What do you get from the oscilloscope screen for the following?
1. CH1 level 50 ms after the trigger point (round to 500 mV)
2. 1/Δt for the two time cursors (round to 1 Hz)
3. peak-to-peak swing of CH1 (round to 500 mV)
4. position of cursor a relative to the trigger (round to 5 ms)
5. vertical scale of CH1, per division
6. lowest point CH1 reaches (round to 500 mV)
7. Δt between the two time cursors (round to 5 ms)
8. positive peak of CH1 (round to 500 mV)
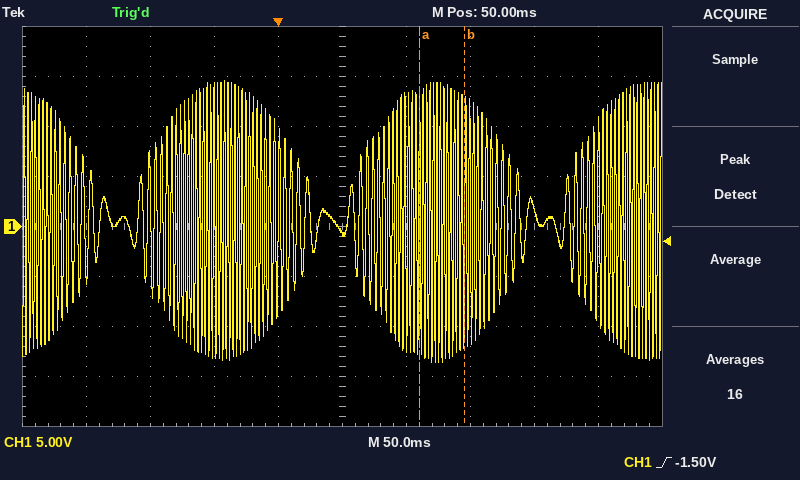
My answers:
-500 mV
29 Hz
28.0 V
+110 ms
5 V
-13.5 V
35 ms
14.5 V
